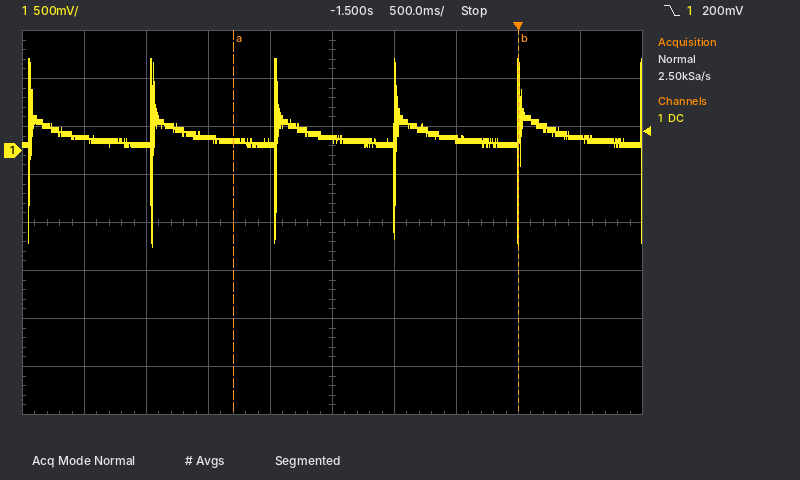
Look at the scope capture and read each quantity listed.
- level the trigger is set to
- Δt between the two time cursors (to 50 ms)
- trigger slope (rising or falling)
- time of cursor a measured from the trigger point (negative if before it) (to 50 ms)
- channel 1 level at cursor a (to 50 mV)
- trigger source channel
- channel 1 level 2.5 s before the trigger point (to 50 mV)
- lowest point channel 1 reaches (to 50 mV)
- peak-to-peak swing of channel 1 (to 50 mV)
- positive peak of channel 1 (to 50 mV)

200 mV
2.30 s
falling
-2.30 s
100 mV
channel 1
150 mV
-1.00 V
1.95 V
950 mV
